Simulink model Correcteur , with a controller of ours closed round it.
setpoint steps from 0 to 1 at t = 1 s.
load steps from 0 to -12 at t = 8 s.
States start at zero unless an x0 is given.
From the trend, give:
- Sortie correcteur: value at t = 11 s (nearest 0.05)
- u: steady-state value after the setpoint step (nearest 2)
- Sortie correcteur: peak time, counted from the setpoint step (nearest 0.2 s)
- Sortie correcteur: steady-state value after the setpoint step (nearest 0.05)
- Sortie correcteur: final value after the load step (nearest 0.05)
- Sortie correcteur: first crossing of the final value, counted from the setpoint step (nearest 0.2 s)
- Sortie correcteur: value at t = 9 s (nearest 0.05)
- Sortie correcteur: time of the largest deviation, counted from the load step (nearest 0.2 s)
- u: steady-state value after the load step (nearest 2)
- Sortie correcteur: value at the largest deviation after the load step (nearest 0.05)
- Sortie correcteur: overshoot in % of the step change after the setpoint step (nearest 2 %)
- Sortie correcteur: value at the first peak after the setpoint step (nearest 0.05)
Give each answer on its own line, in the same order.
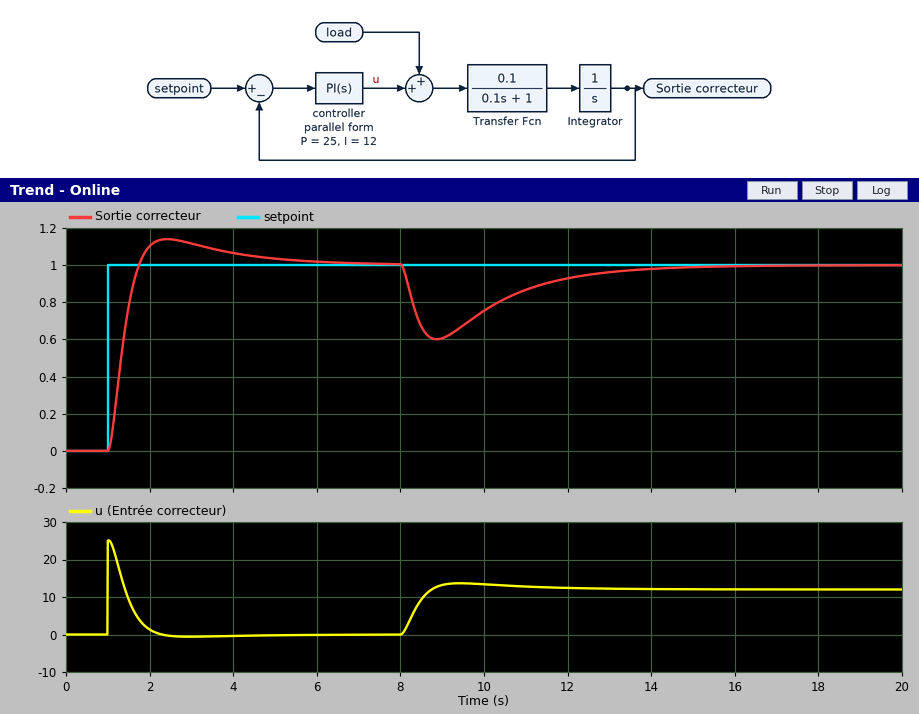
0.85
0
1.4 s
1.00
1.00
0.8 s
0.60
0.8 s
12
0.60
14 %
1.15
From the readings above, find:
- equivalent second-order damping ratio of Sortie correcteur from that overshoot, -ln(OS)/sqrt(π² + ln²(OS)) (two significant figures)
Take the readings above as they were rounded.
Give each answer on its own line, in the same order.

0.53
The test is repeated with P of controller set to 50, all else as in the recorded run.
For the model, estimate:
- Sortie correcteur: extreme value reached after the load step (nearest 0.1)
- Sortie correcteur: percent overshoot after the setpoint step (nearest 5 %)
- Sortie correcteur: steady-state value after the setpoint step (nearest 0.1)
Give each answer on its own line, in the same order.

0.8
10 %
1.0
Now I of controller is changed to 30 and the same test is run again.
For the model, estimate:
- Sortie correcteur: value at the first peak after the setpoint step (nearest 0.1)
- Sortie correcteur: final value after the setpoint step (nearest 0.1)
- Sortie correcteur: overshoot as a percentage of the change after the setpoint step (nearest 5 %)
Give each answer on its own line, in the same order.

1.3
1.0
30 %
